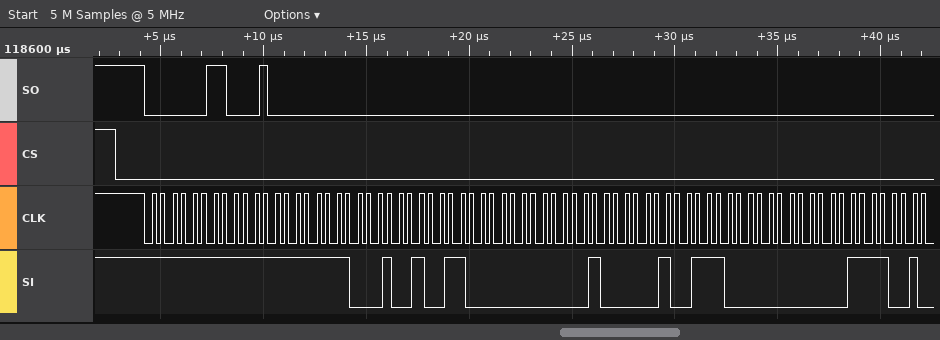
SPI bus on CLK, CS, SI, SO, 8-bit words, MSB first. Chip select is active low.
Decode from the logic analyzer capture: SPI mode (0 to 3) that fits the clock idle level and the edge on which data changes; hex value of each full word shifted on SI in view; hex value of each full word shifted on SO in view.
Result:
3
FF, FF, F1, 26, 00, 10, 27, 00, 0F
03, 10, 00, 00, 00, 00, 00, 00, 00
